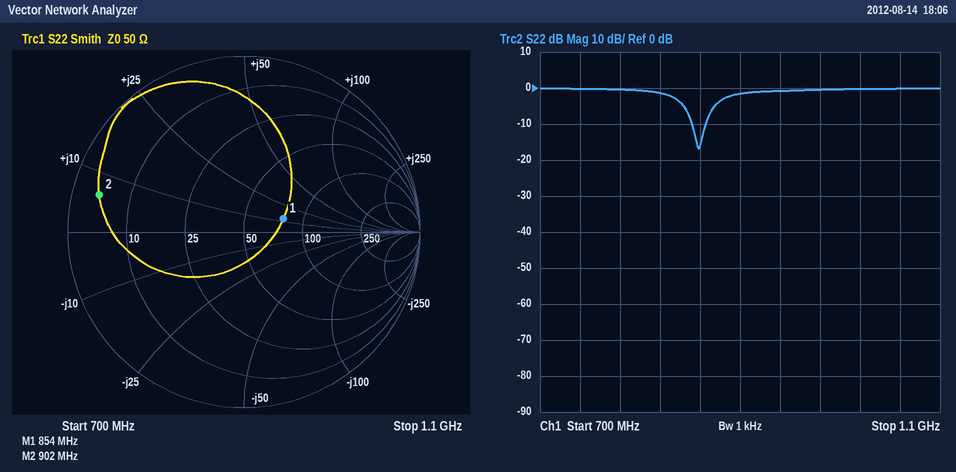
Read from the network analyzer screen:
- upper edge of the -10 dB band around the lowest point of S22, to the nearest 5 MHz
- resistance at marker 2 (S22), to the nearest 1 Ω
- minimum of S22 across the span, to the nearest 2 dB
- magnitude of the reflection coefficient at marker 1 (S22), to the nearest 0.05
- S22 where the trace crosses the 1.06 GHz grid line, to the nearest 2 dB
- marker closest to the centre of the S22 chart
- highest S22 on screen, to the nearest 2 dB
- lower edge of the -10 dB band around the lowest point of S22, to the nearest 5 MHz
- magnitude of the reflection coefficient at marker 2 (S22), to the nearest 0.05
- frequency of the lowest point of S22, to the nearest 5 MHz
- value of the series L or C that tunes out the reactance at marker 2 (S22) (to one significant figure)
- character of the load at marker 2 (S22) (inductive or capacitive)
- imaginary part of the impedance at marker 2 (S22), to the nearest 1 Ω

865 MHz
4 Ω
-16 dB
0.25
0 dB
marker 1
0 dB
850 MHz
0.85
860 MHz
30 pF
inductive
+6 Ω
